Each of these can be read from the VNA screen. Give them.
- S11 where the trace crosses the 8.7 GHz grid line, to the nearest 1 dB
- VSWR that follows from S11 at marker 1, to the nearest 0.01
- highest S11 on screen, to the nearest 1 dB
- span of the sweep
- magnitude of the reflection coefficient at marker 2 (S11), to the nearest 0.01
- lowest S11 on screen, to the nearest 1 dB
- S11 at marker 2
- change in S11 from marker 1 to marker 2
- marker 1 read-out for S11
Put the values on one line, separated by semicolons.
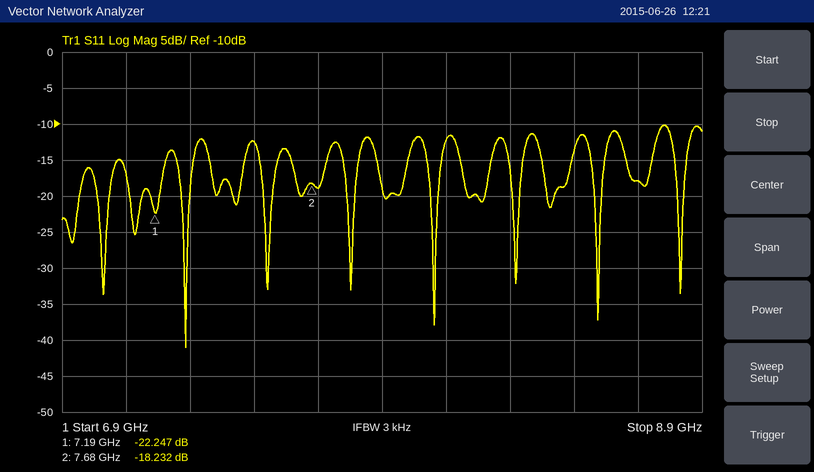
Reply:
-18 dB; 1.17; -10 dB; 2 GHz; 0.12; -41 dB; -18.232 dB; 4.015 dB; -22.247 dB
